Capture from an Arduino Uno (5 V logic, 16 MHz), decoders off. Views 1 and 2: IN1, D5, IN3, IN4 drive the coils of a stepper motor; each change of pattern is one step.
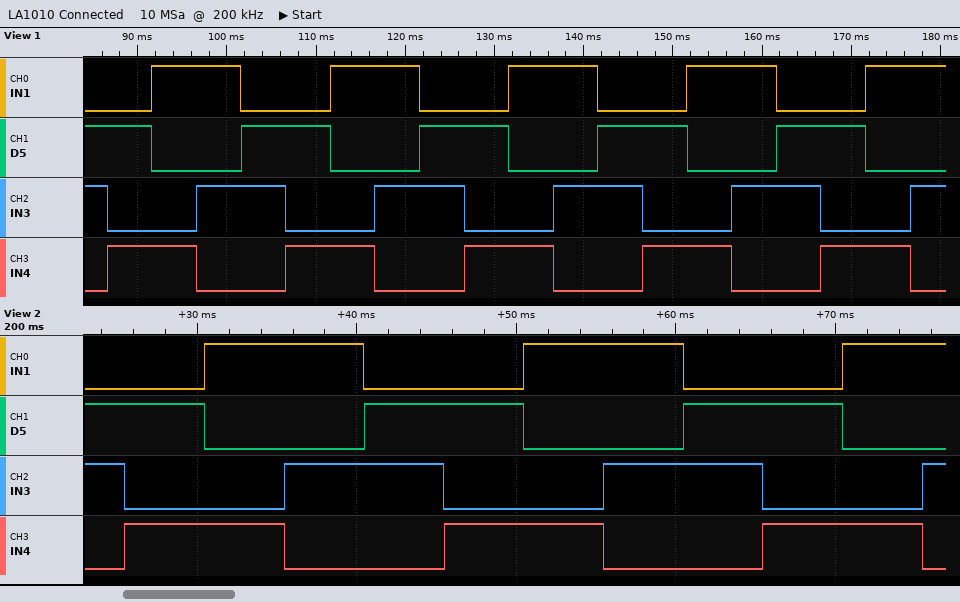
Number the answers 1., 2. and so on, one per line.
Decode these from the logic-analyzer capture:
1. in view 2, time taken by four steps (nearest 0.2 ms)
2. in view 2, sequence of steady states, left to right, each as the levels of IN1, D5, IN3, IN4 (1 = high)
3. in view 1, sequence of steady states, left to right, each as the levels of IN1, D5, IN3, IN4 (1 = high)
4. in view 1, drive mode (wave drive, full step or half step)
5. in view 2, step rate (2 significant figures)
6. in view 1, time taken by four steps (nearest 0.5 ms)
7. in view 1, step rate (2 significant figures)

1. 20.0 ms
2. 0110 0101 1001 1010 0110 0101 1001 1010 0110 0101 1001 1010
3. 0110 0101 1001 1010 0110 0101 1001 1010 0110 0101 1001 1010 0110 0101 1001 1010 0110 0101 1001 1010
4. full step
5. 200 steps/s
6. 20.0 ms
7. 200 steps/s
